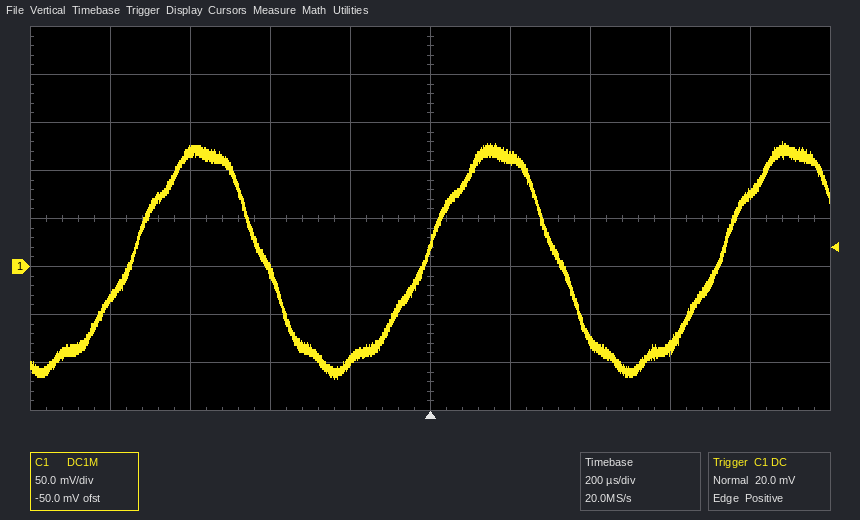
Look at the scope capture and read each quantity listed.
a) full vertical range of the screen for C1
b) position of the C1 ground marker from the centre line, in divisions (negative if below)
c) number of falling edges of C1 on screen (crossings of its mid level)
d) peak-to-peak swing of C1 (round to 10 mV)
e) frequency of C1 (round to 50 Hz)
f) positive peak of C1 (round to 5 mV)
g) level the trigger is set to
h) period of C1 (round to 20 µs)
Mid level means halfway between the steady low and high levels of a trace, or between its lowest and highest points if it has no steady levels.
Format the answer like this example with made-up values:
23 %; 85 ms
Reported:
400 mV; -1.0 div; 2; 250 mV; 1.35 kHz; 130 mV; 20.0 mV; 740 µs
